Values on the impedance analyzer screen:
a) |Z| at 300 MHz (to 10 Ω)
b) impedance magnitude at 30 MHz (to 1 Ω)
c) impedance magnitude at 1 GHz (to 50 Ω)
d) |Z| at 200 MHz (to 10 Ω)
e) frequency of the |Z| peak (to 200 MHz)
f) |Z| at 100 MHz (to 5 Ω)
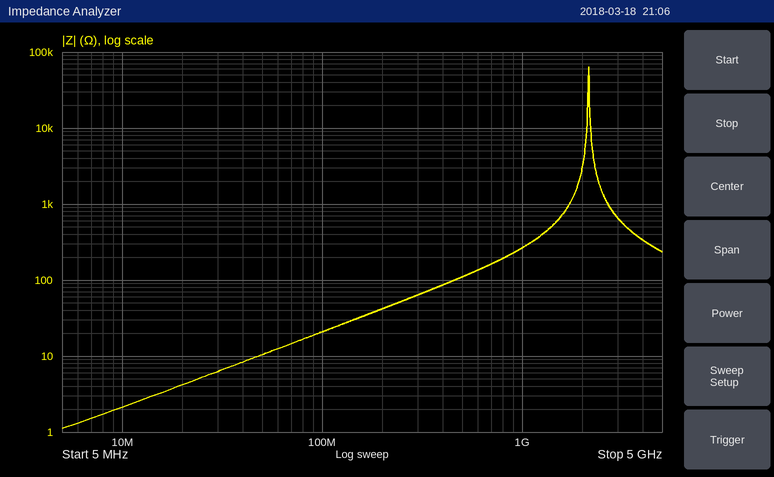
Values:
60 Ω
6 Ω
250 Ω
40 Ω
2.2 GHz
20 Ω
